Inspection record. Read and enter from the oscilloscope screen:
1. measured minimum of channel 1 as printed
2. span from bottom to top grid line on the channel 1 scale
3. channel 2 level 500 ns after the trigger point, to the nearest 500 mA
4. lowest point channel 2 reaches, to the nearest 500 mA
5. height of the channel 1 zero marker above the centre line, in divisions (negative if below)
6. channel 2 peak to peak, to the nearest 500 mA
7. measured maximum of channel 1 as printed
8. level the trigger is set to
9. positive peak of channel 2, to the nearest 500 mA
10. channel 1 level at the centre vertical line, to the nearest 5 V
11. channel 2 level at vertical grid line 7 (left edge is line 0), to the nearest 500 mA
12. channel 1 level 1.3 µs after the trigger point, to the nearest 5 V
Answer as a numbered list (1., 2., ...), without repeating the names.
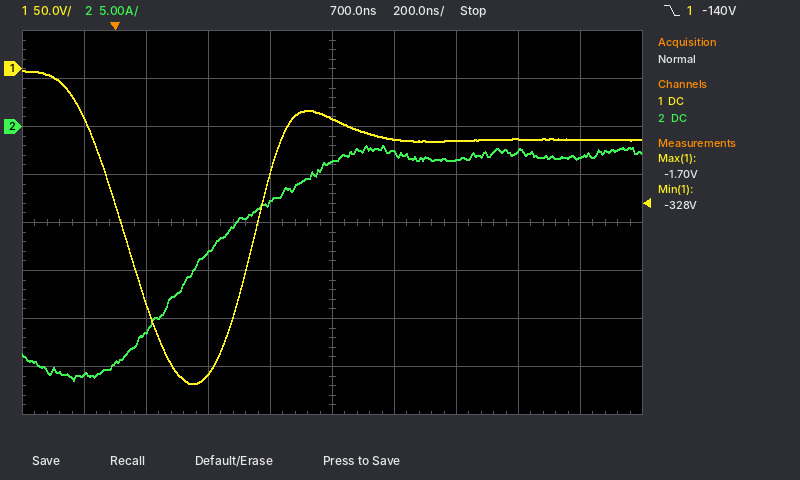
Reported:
1. -328 V
2. 400 V
3. -8.0 A
4. -26.5 A
5. +3.2 div
6. 24.5 A
7. -1.70 V
8. -140 V
9. -2.0 A
10. -50 V
11. -3.5 A
12. -75 V
